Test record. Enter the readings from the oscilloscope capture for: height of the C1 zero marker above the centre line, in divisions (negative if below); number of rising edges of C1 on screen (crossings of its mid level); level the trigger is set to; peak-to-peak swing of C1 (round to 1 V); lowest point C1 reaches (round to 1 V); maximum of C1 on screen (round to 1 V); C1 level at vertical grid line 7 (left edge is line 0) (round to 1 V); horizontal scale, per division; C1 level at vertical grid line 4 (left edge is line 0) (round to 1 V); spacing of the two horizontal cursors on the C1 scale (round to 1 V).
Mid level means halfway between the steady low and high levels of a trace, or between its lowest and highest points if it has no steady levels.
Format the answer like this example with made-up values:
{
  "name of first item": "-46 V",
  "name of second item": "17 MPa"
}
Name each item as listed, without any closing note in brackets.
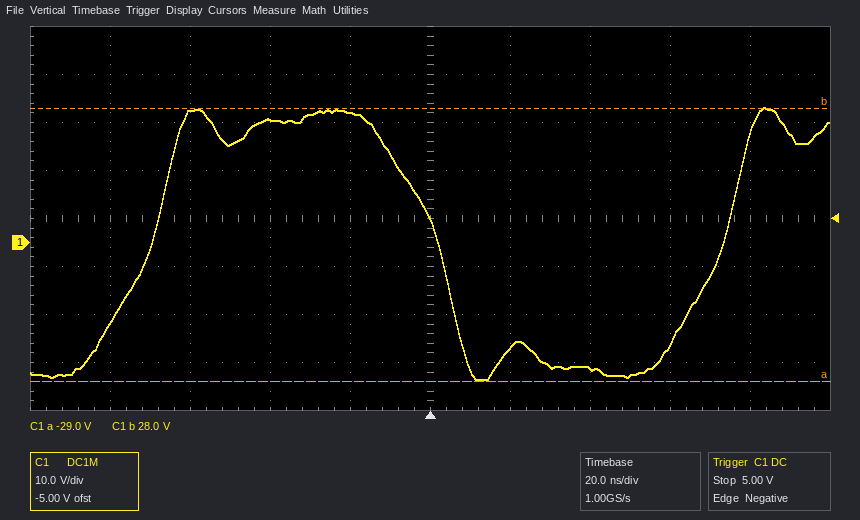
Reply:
{
  "height of the C1 zero marker above the centre line, in divisions": "-0.5 div",
  "number of rising edges of C1 on screen": "2",
  "level the trigger is set to": "5.00 V",
  "peak-to-peak swing of C1": "57 V",
  "lowest point C1 reaches": "-29 V",
  "maximum of C1 on screen": "28 V",
  "C1 level at vertical grid line 7 (left edge is line 0)": "-26 V",
  "horizontal scale, per division": "20 ns",
  "C1 level at vertical grid line 4 (left edge is line 0)": "27 V",
  "spacing of the two horizontal cursors on the C1 scale": "57 V"
}
